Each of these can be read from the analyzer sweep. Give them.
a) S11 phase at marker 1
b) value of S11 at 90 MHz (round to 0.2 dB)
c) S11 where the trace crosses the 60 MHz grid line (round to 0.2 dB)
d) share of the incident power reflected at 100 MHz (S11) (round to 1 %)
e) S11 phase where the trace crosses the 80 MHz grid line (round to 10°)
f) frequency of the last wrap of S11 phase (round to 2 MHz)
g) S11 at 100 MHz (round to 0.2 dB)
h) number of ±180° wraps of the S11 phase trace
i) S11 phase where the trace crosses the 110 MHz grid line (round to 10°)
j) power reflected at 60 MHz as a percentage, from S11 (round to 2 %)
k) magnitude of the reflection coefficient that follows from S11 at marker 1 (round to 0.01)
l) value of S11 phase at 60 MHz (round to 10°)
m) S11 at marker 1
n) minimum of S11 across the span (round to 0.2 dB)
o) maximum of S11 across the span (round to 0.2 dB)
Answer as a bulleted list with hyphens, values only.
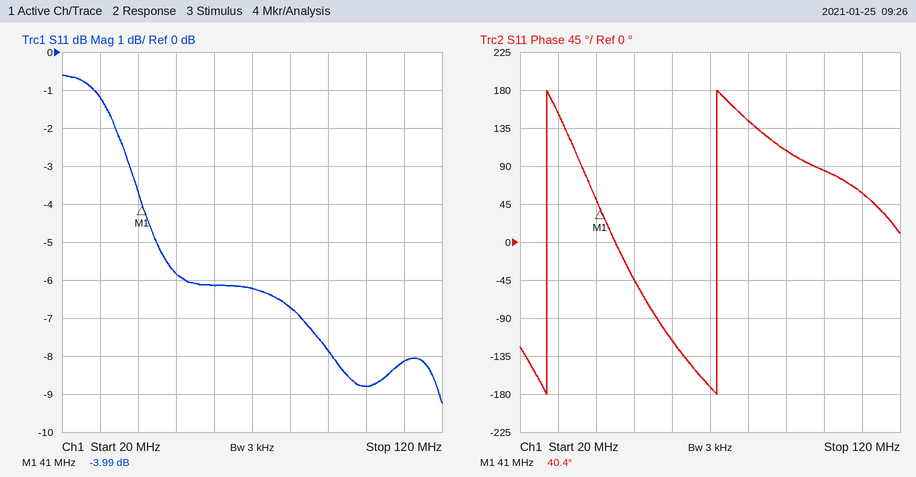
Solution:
- 40.4°
- -7.8 dB
- -6.2 dB
- 13 %
- 140°
- 72 MHz
- -8.8 dB
- 2
- 60°
- 24 %
- 0.63
- -120°
- -3.99 dB
- -9.2 dB
- -0.6 dB
